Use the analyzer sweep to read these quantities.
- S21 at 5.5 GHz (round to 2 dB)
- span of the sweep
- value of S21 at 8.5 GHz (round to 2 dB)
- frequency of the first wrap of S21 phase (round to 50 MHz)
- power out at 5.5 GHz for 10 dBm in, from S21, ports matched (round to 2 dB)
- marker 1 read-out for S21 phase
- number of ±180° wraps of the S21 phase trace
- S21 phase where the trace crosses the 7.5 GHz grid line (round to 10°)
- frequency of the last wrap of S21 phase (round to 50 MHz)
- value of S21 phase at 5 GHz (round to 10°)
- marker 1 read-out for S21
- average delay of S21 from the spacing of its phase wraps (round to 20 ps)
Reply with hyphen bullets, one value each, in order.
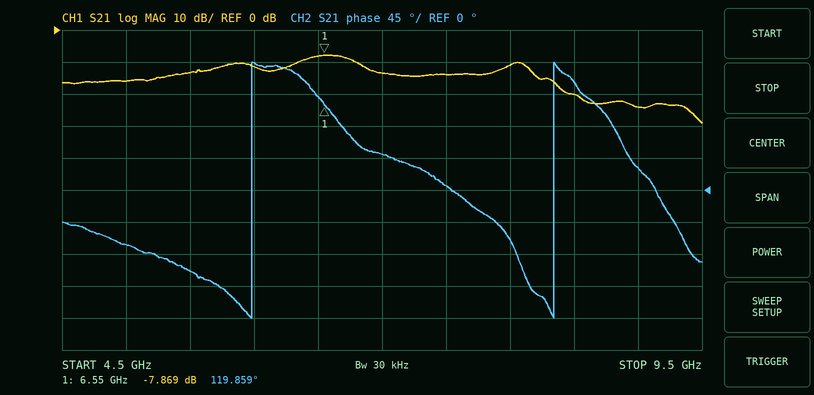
- -14 dB
- 5 GHz
- -20 dB
- 6.00 GHz
- -4 dBm
- 119.859°
- 2
- 10°
- 8.35 GHz
- -80°
- -7.869 dB
- 420 ps
